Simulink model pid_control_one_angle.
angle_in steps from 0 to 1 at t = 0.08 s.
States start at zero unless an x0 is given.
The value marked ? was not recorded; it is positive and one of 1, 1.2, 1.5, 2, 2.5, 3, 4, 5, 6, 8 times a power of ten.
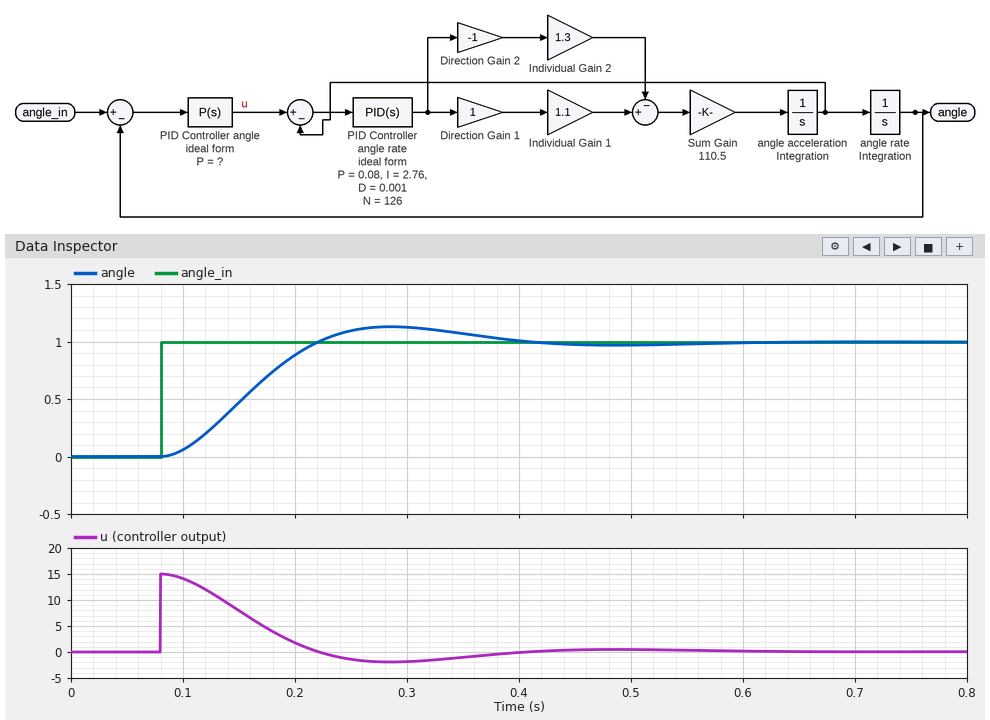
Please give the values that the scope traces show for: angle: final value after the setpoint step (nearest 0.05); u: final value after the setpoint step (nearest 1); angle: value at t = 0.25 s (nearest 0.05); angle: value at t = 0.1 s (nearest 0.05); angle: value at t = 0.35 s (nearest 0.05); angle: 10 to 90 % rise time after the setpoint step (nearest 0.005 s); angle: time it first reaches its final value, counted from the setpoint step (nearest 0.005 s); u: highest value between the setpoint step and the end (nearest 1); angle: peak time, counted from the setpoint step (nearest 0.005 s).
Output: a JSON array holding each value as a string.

["1.00", "0", "1.10", "0.05", "1.05", "0.095 s", "0.140 s", "15", "0.205 s"]
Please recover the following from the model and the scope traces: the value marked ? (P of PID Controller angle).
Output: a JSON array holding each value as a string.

["15"]
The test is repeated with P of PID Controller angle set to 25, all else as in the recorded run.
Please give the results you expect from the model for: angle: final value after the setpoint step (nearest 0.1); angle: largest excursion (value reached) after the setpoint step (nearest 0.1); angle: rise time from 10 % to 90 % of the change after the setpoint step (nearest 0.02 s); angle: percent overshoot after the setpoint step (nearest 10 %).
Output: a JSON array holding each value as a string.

["1.0", "1.2", "0.06 s", "20 %"]
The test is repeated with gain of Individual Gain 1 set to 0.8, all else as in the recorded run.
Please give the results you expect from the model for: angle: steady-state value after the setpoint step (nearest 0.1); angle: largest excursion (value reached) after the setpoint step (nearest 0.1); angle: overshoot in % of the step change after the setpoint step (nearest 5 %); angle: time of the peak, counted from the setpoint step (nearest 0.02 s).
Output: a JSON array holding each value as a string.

["1.0", "1.2", "15 %", "0.22 s"]
